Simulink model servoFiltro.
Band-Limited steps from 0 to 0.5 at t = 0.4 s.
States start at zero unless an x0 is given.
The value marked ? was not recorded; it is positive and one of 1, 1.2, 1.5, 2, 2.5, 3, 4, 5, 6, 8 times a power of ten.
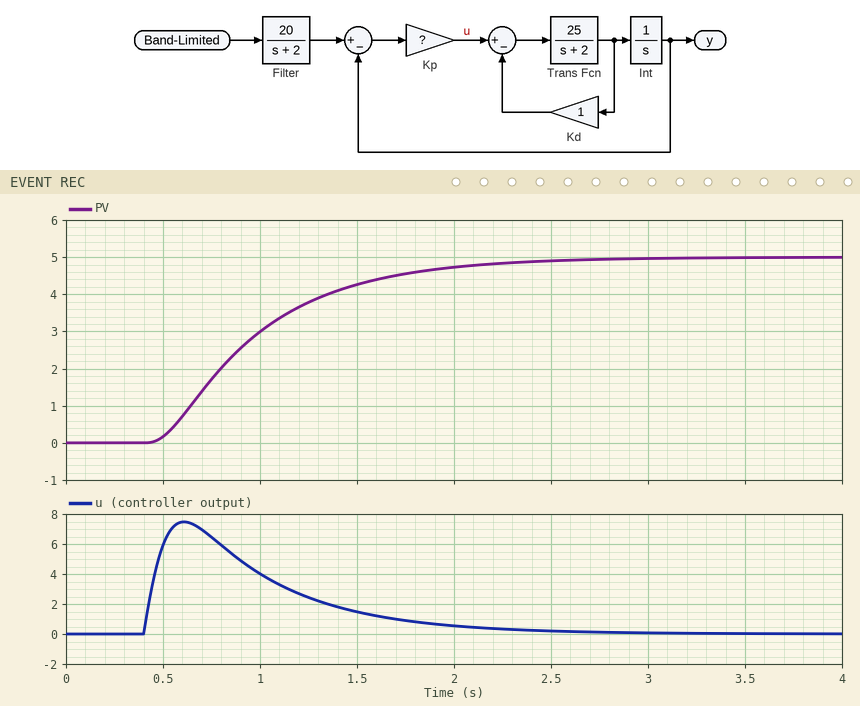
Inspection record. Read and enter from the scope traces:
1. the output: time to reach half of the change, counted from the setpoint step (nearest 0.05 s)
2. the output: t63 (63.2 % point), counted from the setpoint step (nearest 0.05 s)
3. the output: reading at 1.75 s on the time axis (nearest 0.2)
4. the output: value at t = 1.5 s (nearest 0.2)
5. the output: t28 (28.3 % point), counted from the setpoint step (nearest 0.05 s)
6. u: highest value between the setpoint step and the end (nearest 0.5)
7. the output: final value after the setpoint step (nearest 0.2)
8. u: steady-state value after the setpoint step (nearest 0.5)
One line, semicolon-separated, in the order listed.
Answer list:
0.50 s; 0.65 s; 4.6; 4.2; 0.30 s; 7.5; 5.0; 0.0
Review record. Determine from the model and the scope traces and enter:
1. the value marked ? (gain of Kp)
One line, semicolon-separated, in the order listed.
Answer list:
8
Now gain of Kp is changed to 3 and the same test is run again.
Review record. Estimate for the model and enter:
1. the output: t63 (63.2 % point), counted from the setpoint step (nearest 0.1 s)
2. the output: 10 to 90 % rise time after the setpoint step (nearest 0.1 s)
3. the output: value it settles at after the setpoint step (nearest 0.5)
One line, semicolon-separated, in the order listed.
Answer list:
0.9 s; 1.4 s; 5.0
